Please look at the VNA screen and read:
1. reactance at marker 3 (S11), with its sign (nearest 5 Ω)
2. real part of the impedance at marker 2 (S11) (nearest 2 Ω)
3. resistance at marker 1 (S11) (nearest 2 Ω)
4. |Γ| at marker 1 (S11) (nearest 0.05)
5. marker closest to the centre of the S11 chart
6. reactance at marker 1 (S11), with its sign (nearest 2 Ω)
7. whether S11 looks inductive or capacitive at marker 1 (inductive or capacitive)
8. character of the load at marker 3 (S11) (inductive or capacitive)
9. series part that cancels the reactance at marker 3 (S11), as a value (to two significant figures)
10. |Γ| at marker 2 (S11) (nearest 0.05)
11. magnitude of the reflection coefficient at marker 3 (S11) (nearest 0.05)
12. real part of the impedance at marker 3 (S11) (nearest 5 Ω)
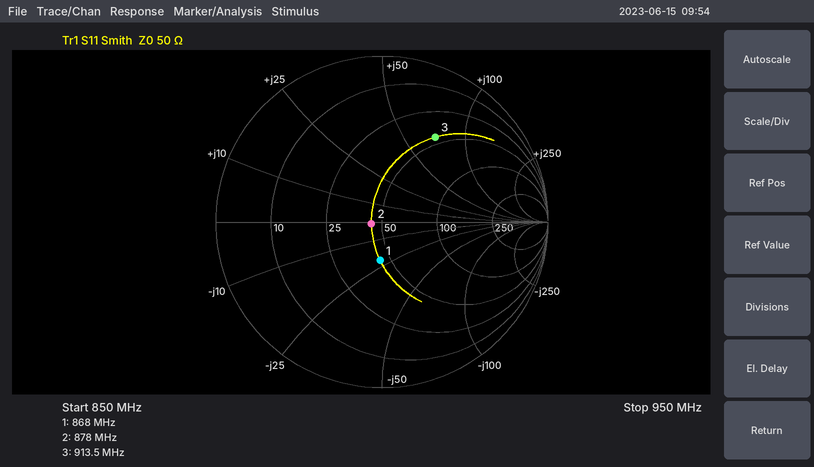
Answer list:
+70 Ω
44 Ω
44 Ω
0.25
marker 2
-22 Ω
capacitive
inductive
2.5 pF
0.05
0.60
45 Ω
